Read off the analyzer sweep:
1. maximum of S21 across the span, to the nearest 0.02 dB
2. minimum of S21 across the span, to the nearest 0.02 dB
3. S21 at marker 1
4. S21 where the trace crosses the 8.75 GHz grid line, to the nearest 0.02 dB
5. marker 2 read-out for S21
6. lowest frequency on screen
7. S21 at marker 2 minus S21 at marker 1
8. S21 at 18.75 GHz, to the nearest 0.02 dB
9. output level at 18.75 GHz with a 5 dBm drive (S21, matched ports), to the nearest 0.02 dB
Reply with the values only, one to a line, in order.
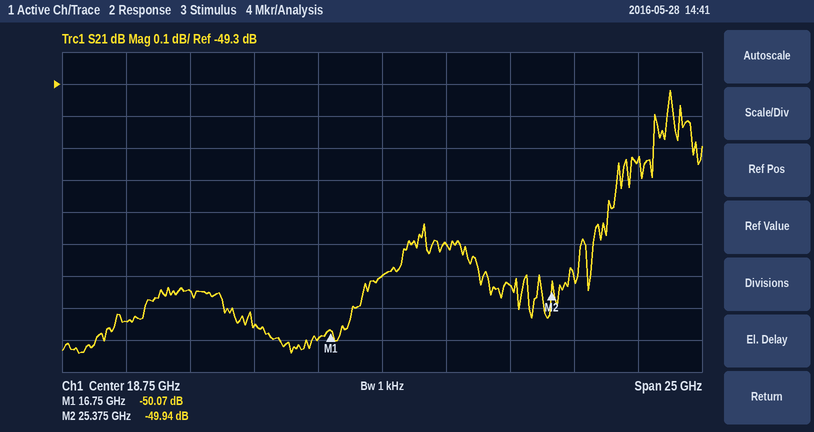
-49.32 dB
-50.14 dB
-50.07 dB
-50.04 dB
-49.94 dB
6.25 GHz
0.13 dB
-49.90 dB
-44.90 dBm
